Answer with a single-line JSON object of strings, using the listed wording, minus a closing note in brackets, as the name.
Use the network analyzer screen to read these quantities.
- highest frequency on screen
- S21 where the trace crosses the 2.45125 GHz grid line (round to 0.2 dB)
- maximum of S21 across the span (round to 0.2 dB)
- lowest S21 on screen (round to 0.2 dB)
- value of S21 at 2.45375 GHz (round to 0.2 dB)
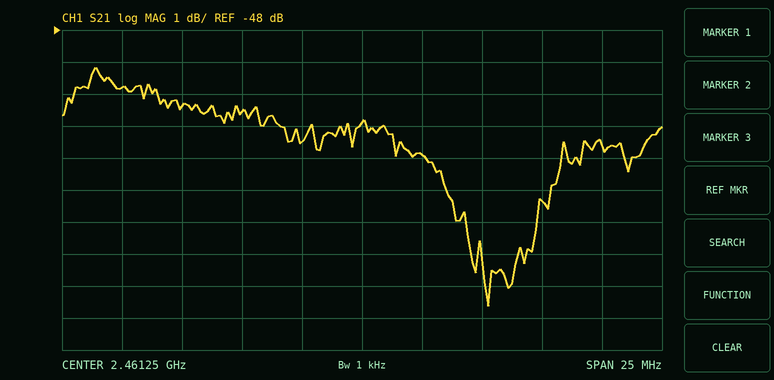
{"highest frequency on screen": "2.47375 GHz", "S21 where the trace crosses the 2.45125 GHz grid line": "-49.8 dB", "maximum of S21 across the span": "-49.2 dB", "lowest S21 on screen": "-56.6 dB", "value of S21 at 2.45375 GHz": "-50.4 dB"}
